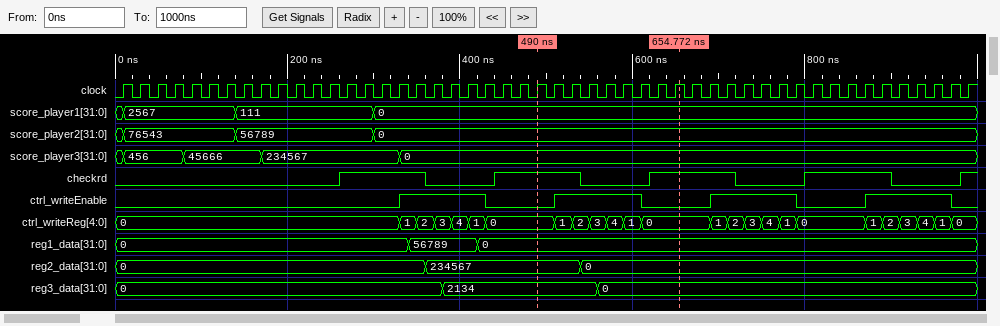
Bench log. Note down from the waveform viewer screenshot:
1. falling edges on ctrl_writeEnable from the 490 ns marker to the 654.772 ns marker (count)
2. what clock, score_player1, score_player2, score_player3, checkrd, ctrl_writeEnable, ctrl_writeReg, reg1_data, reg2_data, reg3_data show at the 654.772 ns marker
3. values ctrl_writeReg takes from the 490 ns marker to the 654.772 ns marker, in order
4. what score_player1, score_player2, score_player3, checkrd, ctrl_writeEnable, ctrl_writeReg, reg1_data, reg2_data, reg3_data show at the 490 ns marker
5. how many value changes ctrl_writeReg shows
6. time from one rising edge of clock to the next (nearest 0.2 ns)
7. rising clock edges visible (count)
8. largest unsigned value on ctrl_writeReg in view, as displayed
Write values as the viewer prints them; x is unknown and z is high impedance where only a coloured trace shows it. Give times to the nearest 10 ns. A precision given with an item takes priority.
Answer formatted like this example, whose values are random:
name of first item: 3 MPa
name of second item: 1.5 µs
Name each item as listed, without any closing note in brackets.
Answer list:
falling edges on ctrl_writeEnable from the 490 ns marker to the 654.772 ns marker: 1
what clock, score_player1, score_player2, score_player3, checkrd, ctrl_writeEnable, ctrl_writeReg, reg1_data, reg2_data, reg3_data show at the 654.772 ns marker: clock=1, score_player1=0, score_player2=0, score_player3=0, checkrd=1, ctrl_writeEnable=0, ctrl_writeReg=0, reg1_data=0, reg2_data=0, reg3_data=0
values ctrl_writeReg takes from the 490 ns marker to the 654.772 ns marker, in order: 0, 1, 2, 3, 4, 1, 0
what score_player1, score_player2, score_player3, checkrd, ctrl_writeEnable, ctrl_writeReg, reg1_data, reg2_data, reg3_data show at the 490 ns marker: score_player1=0, score_player2=0, score_player3=0, checkrd=1, ctrl_writeEnable=0, ctrl_writeReg=0, reg1_data=0, reg2_data=234567, reg3_data=2134
how many value changes ctrl_writeReg shows: 24
time from one rising edge of clock to the next: 20 ns
rising clock edges visible: 50
largest unsigned value on ctrl_writeReg in view, as displayed: 4
